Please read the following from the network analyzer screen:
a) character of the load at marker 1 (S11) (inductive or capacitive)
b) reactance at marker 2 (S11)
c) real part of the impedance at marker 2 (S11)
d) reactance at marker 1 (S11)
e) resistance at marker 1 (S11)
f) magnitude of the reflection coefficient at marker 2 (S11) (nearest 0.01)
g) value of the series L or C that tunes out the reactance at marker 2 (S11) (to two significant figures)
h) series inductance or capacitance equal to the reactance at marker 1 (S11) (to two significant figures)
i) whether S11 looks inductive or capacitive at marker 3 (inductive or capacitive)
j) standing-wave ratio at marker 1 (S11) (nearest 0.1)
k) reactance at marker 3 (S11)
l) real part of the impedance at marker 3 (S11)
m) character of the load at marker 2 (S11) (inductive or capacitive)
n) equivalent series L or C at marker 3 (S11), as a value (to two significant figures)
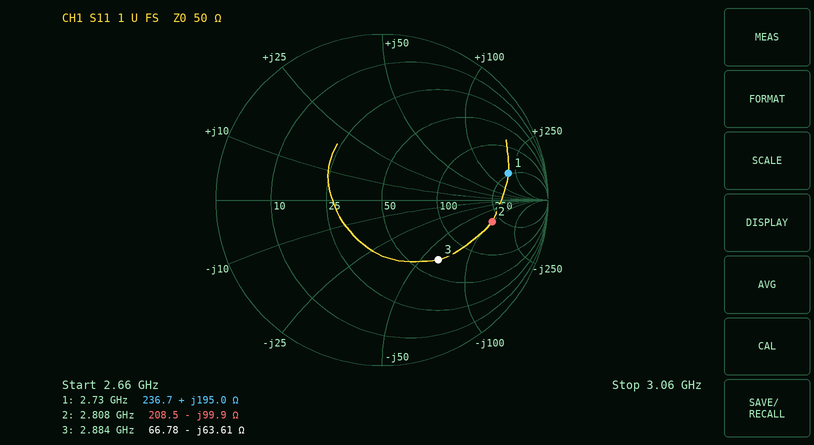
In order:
inductive
-99.9 Ω
208.5 Ω
+195.0 Ω
236.7 Ω
0.68
5.7 nH
11 nH
capacitive
8.0
-63.61 Ω
66.78 Ω
capacitive
870 fF
